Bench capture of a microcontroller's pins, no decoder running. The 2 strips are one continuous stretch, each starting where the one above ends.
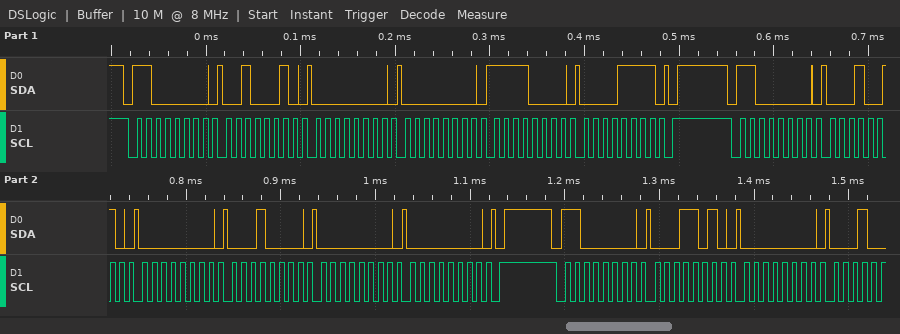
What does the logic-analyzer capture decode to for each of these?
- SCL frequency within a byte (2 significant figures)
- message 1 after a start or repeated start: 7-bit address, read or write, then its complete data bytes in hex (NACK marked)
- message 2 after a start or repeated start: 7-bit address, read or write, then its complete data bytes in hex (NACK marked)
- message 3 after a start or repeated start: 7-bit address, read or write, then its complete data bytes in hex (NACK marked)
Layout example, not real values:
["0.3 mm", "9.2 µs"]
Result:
["100 kHz", "0x60 write: 22 00 00 F0 0F", "0x60 write: 12 00 10 00 00", "0x60 write: 1A 00"]
